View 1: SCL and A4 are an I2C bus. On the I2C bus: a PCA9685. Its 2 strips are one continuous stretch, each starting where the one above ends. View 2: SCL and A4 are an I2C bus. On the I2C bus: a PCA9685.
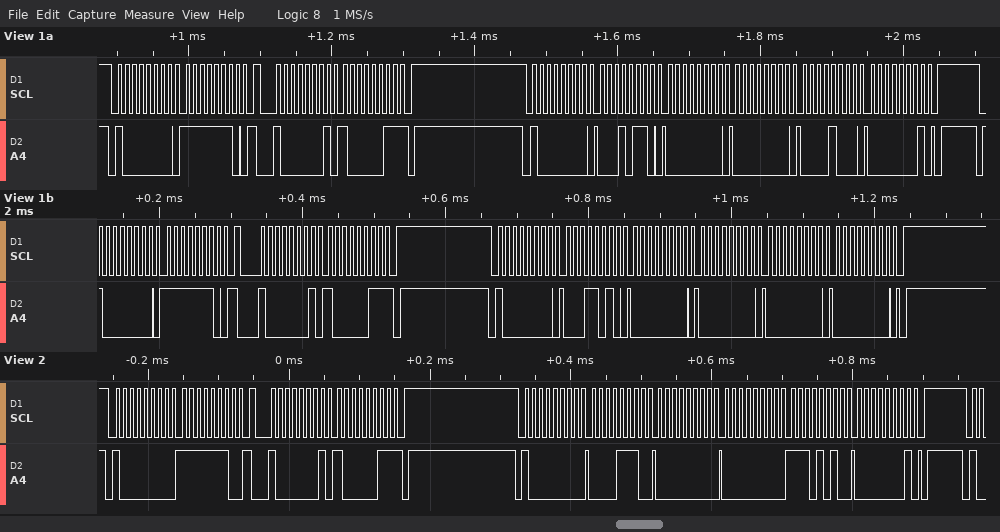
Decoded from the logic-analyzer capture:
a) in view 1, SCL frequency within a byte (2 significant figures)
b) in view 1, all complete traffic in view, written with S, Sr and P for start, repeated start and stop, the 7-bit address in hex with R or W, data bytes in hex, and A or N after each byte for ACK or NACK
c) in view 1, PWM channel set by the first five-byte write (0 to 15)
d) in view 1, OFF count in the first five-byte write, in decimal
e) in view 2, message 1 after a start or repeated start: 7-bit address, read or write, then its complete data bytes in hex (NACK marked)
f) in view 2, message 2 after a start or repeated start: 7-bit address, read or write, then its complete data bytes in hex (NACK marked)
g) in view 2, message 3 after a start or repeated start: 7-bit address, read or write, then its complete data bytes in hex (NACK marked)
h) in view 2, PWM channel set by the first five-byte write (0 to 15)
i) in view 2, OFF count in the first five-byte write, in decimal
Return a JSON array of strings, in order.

["100 kHz", "S 40W A FE A Sr 40R A 83 N P S 40W A 16 A 00 A 00 A 08 A 01 A P S 40W A FE A Sr 40R A 83 N P S 40W A 1A A 00 A 00 A 00 A 00 A P", "4", "264", "0x40 write: FE", "0x40 read: 83 NACK", "0x40 write: 0E 00 00 EA 01", "2", "490"]
